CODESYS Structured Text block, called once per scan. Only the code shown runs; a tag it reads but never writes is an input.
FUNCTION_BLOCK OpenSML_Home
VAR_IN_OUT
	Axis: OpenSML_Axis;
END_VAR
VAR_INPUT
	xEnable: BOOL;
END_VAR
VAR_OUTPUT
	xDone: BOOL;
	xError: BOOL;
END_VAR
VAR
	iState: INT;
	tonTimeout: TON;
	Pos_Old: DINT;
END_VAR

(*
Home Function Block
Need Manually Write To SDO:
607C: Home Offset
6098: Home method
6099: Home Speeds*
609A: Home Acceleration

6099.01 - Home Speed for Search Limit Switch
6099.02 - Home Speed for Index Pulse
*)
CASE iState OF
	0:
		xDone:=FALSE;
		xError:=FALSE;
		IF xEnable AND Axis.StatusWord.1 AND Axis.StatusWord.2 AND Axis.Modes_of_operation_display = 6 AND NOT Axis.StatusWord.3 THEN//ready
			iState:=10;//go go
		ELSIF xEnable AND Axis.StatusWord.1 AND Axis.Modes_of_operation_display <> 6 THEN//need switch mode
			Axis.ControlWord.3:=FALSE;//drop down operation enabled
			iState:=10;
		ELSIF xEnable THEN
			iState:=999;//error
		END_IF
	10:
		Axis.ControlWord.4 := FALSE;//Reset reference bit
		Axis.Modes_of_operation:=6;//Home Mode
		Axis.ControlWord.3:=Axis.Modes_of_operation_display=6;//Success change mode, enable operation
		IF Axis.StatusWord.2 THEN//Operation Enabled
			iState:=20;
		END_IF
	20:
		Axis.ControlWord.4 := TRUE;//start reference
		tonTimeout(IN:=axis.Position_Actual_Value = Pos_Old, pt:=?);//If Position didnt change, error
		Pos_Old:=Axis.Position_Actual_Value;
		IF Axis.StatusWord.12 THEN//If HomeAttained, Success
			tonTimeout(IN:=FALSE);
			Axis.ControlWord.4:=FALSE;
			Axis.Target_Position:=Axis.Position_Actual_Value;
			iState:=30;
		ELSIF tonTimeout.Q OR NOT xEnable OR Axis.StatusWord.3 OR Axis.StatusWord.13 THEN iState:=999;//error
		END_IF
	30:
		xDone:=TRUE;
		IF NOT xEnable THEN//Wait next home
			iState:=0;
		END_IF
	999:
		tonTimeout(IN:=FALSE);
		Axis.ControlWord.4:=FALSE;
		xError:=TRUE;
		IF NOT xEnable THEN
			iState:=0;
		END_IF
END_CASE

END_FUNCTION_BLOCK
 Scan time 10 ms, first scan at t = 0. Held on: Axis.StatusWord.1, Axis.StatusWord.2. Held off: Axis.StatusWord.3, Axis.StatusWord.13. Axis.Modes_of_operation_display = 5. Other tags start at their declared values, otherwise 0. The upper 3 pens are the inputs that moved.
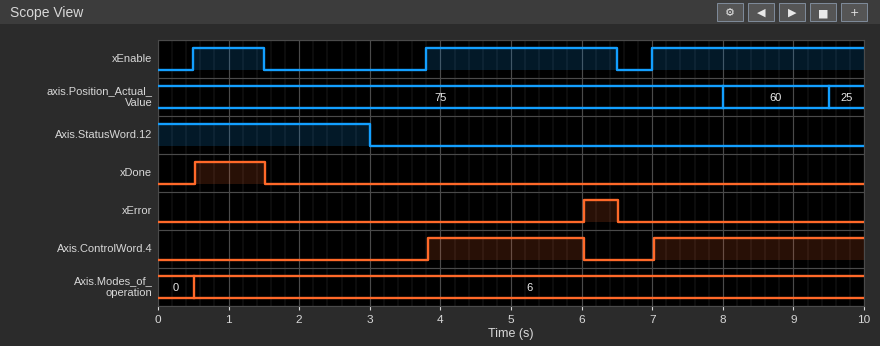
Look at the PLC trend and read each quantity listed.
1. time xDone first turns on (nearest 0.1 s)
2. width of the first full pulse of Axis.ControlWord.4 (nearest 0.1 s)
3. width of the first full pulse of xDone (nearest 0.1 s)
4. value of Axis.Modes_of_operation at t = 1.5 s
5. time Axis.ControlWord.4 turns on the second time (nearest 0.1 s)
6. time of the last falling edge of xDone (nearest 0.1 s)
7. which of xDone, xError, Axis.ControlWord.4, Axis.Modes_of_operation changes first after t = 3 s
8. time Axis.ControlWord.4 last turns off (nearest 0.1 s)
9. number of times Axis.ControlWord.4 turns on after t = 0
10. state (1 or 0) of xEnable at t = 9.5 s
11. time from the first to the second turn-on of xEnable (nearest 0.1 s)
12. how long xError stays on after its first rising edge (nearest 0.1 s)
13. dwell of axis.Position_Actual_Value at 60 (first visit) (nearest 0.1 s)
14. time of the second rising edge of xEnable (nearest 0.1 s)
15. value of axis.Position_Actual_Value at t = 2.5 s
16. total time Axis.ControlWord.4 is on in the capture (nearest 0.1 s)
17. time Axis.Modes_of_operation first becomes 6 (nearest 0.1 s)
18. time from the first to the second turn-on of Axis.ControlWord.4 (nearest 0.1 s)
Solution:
0.5 s
2.2 s
1.0 s
6
7.0 s
1.5 s
Axis.ControlWord.4
6.0 s
2
1
3.3 s
0.5 s
1.5 s
3.8 s
75
5.2 s
0.5 s
3.2 s
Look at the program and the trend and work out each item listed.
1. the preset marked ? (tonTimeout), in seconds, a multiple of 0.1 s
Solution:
2.2 s
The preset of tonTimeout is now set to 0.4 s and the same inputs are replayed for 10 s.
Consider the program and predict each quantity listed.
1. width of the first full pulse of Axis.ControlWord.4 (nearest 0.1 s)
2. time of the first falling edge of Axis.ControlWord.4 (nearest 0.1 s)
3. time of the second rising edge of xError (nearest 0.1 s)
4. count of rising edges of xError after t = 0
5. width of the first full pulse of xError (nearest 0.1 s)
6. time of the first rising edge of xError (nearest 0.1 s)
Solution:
0.4 s
4.2 s
7.4 s
2
2.3 s
4.2 s
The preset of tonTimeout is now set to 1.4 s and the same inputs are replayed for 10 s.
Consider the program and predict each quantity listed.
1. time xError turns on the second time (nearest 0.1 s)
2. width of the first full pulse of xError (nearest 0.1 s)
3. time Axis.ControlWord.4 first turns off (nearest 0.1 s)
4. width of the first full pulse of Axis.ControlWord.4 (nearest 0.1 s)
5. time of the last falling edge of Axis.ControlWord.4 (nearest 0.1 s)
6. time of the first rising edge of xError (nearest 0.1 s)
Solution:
9.4 s
1.3 s
5.2 s
1.4 s
9.4 s
5.2 s
